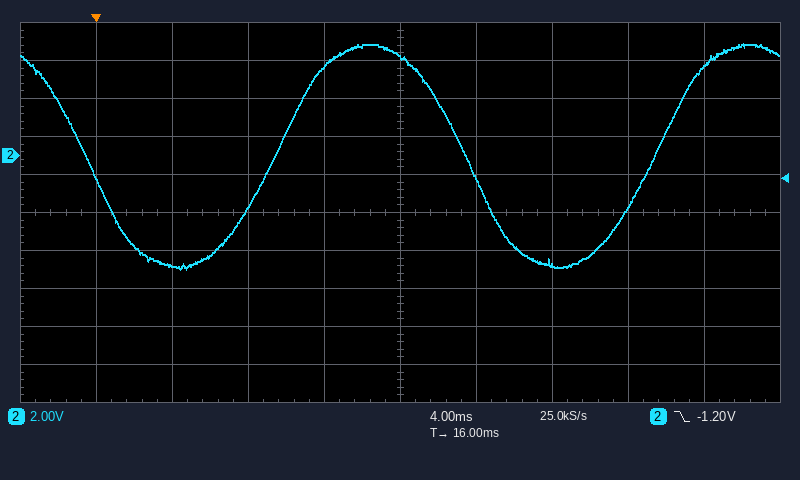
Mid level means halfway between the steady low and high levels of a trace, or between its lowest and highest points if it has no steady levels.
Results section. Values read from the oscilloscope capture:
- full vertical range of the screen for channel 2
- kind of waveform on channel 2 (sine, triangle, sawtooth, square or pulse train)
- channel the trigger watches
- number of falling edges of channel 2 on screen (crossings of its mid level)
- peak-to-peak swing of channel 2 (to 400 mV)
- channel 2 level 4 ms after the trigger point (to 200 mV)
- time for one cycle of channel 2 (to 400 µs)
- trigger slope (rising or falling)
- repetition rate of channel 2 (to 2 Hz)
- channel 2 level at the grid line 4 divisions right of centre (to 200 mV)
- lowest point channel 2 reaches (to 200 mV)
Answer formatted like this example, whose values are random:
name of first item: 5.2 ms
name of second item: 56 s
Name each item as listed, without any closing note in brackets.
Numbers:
full vertical range of the screen for channel 2: 20 V
kind of waveform on channel 2: sine
channel the trigger watches: channel 2
number of falling edges of channel 2 on screen: 2
peak-to-peak swing of channel 2: 12.0 V
channel 2 level 4 ms after the trigger point: -5.8 V
time for one cycle of channel 2: 20.0 ms
trigger slope: falling
repetition rate of channel 2: 50 Hz
channel 2 level at the grid line 4 divisions right of centre: 4.6 V
lowest point channel 2 reaches: -6.0 V
